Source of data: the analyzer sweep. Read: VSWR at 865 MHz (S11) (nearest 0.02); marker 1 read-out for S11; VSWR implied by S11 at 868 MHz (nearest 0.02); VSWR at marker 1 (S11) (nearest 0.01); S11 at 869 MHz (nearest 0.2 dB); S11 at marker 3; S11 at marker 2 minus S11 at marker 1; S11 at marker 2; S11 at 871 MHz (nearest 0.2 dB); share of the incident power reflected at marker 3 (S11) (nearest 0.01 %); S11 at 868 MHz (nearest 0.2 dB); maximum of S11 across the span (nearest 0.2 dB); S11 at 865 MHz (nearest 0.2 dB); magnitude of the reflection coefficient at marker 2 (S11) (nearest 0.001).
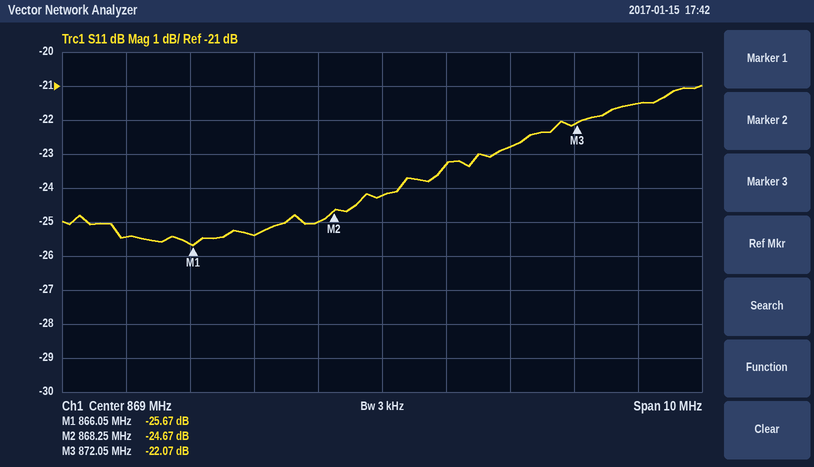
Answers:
1.12
-25.67 dB
1.12
1.11
-24.2 dB
-22.07 dB
1.00 dB
-24.67 dB
-22.8 dB
0.62 %
-25.0 dB
-21.0 dB
-25.4 dB
0.058
